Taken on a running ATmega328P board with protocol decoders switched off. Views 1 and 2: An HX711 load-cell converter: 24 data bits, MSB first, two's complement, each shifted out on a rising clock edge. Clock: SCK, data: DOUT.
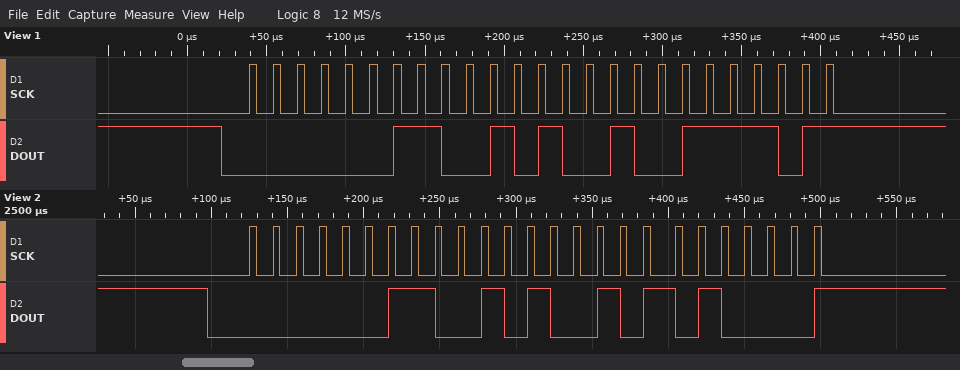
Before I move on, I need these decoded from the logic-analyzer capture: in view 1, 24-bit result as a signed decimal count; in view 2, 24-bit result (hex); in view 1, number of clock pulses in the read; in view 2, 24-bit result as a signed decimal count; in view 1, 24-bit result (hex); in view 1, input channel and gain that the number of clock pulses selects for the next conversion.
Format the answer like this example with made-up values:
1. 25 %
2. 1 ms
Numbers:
1. 207165
2. 0x032950
3. 25
4. 207184
5. 0x03293D
6. channel A, gain 128
